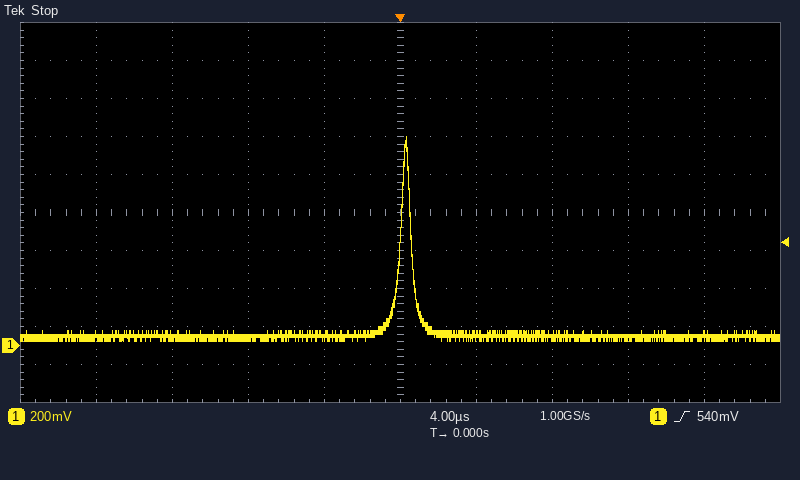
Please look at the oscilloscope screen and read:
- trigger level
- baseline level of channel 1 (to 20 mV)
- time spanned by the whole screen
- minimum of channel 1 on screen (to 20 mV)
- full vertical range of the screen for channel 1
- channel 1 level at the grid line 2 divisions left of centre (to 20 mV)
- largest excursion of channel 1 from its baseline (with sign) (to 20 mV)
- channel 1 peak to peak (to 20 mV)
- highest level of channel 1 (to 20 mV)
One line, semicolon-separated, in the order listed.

540 mV; 40 mV; 40 µs; 20 mV; 2 V; 40 mV; +1.06 V; 1.08 V; 1.10 V
